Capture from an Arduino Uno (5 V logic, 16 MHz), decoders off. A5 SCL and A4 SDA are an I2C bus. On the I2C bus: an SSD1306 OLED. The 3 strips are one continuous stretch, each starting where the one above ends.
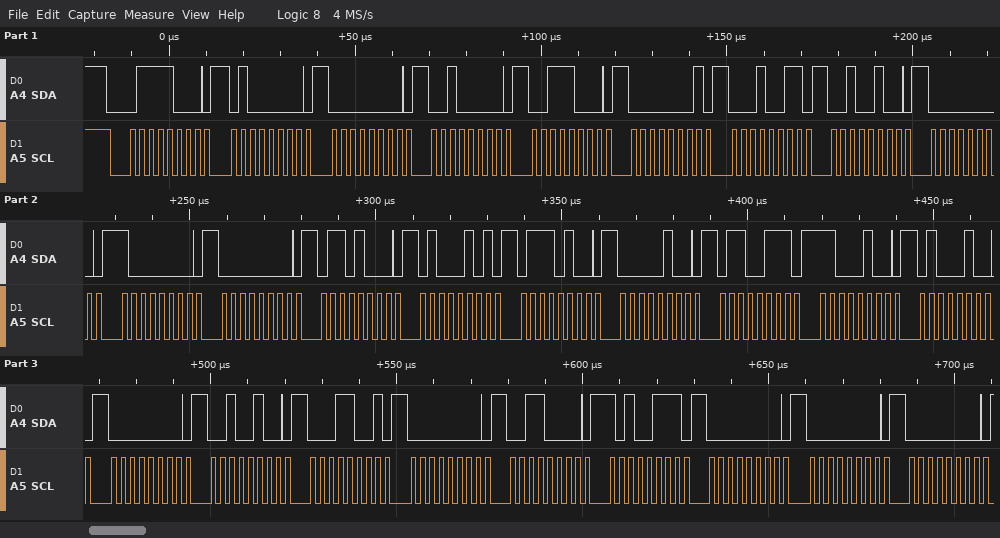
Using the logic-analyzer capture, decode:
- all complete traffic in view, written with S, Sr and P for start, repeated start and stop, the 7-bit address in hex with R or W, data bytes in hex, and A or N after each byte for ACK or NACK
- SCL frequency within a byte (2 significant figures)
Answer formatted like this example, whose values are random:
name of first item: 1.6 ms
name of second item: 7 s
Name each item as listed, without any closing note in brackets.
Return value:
all complete traffic in view, written with S, Sr and P for start, repeated start and stop, the 7-bit address in hex with R or W, data bytes in hex, and A or N after each byte for ACK or NACK: S 3CW A 40 A 00 A 20 A 38 A 01 A 13 A 24 A 00 A 80 A 00 A 68 A 45 A 74 A 04 A 67 A C4 A 44 A 00 A 24 A 19 A 00 A 30 A A7 A 00 A 00 A 00 A
SCL frequency within a byte: 400 kHz
